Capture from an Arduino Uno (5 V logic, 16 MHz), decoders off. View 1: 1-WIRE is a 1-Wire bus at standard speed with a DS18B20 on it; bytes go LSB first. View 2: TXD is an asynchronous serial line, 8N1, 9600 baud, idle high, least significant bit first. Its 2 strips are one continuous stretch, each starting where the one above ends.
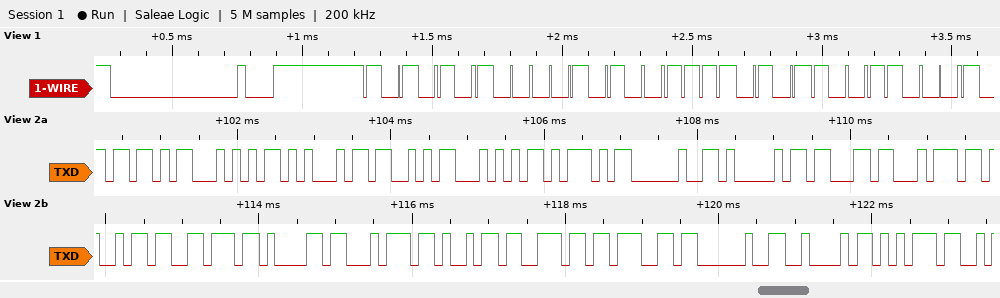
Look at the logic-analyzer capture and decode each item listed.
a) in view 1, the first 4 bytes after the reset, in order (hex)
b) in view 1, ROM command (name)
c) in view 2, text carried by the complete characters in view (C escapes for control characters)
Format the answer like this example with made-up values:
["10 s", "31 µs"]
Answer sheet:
["55 28 AF 19", "Match ROM", "\"[TEST] Activating Bu\""]
